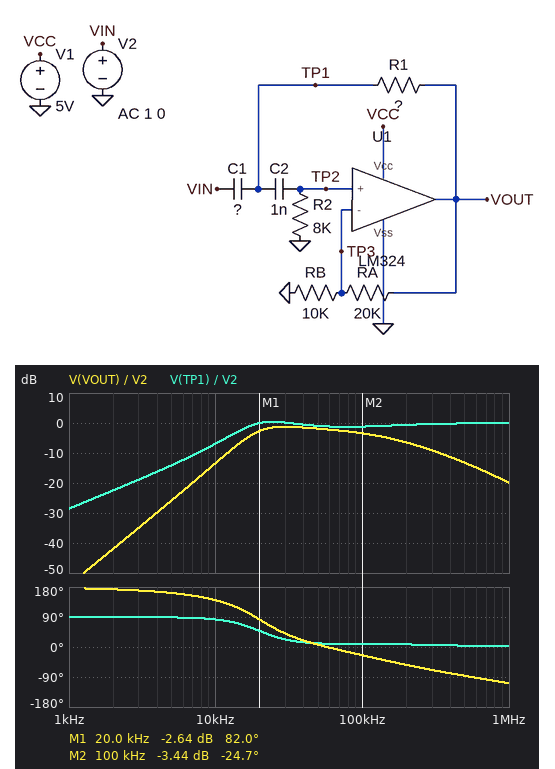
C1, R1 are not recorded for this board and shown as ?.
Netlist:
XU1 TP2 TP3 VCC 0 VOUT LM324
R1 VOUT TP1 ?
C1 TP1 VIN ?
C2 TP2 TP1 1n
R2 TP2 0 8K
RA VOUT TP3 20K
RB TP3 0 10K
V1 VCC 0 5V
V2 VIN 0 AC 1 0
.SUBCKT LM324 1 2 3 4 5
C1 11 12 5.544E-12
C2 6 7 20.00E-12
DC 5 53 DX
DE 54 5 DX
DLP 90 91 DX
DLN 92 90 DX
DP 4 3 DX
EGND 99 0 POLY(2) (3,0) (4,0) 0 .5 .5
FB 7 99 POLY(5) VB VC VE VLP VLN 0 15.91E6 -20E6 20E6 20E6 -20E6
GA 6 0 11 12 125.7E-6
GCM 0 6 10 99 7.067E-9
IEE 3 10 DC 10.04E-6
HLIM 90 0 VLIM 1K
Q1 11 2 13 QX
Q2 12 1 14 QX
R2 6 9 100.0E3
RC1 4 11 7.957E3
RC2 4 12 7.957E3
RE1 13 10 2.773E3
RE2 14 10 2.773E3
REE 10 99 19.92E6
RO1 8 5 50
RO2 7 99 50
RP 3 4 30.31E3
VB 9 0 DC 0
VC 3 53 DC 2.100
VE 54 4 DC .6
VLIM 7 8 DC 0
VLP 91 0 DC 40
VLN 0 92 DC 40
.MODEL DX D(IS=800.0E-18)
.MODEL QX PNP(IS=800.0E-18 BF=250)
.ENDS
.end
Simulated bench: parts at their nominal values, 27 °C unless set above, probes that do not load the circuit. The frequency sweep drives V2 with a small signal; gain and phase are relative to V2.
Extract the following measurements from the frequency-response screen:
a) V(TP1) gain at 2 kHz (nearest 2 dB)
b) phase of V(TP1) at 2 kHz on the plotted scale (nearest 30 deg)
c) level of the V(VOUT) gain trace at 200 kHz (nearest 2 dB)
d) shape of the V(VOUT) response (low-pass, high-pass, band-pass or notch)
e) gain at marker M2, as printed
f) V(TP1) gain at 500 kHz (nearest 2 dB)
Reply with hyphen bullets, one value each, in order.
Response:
- -22 dB
- 90 deg
- -6 dB
- band-pass
- -3.44 dB
- 0 dB
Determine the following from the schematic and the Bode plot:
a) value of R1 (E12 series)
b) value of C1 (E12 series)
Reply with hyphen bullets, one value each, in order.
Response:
- 2.7 kΩ
- 2.2 nF
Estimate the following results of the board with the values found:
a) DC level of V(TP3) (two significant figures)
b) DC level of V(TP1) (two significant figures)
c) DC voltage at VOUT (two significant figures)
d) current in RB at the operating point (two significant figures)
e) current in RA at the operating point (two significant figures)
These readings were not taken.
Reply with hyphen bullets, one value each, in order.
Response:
- 16 mV
- 47 mV
- 47 mV
- 1.6 µA
- 1.6 µA
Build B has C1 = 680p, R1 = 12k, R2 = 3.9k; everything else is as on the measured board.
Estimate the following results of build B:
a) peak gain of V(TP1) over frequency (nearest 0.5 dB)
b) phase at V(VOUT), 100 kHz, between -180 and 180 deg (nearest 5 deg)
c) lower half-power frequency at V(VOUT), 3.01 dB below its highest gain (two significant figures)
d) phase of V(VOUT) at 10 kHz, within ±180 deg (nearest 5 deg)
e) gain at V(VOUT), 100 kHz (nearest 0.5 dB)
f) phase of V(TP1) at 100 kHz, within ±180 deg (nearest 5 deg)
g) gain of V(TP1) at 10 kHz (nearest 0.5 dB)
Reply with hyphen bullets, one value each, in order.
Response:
- 0 dB
- 0 deg
- 39 kHz
- 120 deg
- -5.5 dB
- 25 deg
- -9.0 dB
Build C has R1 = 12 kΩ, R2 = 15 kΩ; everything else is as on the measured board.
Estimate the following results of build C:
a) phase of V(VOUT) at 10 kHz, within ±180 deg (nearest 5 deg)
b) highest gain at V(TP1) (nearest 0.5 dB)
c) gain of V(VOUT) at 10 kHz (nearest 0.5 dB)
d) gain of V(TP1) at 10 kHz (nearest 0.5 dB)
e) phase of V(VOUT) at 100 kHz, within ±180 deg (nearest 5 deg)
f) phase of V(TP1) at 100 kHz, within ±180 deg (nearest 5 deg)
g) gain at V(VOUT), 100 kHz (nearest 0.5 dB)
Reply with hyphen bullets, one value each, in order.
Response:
- 70 deg
- 0 dB
- -3.5 dB
- -0.5 dB
- -35 deg
- 5 deg
- -2.5 dB
